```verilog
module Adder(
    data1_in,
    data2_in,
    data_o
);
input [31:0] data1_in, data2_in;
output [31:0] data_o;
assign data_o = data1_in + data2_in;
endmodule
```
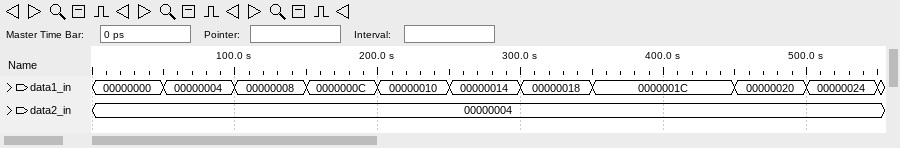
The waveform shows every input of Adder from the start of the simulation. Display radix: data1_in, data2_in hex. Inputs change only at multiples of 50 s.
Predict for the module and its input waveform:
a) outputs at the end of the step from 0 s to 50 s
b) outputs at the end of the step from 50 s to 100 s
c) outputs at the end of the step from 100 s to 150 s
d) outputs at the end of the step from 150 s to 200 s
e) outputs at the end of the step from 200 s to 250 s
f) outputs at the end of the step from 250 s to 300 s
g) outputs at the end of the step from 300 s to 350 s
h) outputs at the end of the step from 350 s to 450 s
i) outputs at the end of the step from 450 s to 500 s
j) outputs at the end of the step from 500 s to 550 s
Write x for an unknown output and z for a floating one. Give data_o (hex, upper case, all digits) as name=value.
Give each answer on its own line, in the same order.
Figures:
data_o=00000004
data_o=00000008
data_o=0000000C
data_o=00000010
data_o=00000014
data_o=00000018
data_o=0000001C
data_o=00000020
data_o=00000024
data_o=00000028
